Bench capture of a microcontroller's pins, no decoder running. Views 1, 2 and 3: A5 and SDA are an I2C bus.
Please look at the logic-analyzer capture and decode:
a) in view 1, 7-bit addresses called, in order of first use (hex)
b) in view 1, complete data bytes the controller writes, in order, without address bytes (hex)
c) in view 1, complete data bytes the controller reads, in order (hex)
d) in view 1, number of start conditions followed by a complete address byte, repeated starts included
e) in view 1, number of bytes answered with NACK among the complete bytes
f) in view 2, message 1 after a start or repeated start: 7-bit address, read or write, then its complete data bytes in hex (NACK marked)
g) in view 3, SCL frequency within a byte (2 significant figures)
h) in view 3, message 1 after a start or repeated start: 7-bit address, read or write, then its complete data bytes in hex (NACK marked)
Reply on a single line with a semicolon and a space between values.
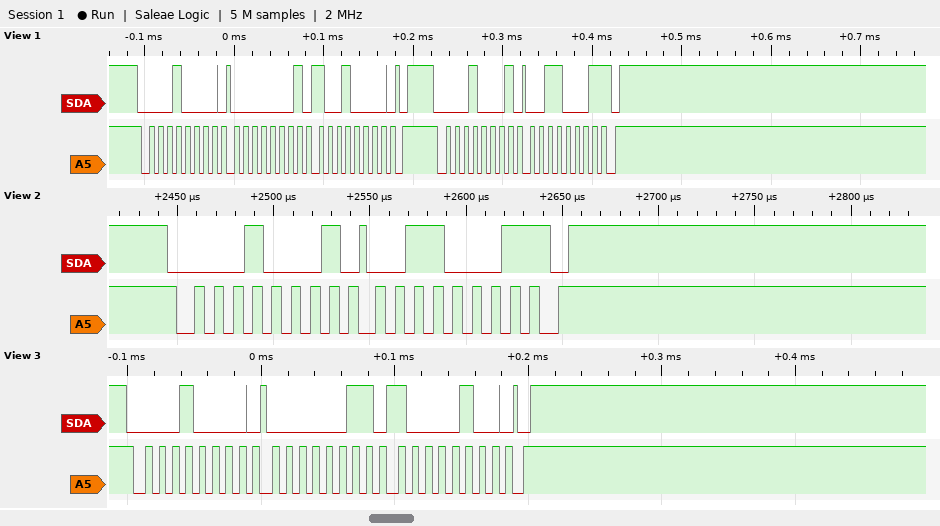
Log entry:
0x08; 01 90; 31; 2; 1; 0x08 read: 31 NACK; 100 kHz; 0x08 write: 03 84
